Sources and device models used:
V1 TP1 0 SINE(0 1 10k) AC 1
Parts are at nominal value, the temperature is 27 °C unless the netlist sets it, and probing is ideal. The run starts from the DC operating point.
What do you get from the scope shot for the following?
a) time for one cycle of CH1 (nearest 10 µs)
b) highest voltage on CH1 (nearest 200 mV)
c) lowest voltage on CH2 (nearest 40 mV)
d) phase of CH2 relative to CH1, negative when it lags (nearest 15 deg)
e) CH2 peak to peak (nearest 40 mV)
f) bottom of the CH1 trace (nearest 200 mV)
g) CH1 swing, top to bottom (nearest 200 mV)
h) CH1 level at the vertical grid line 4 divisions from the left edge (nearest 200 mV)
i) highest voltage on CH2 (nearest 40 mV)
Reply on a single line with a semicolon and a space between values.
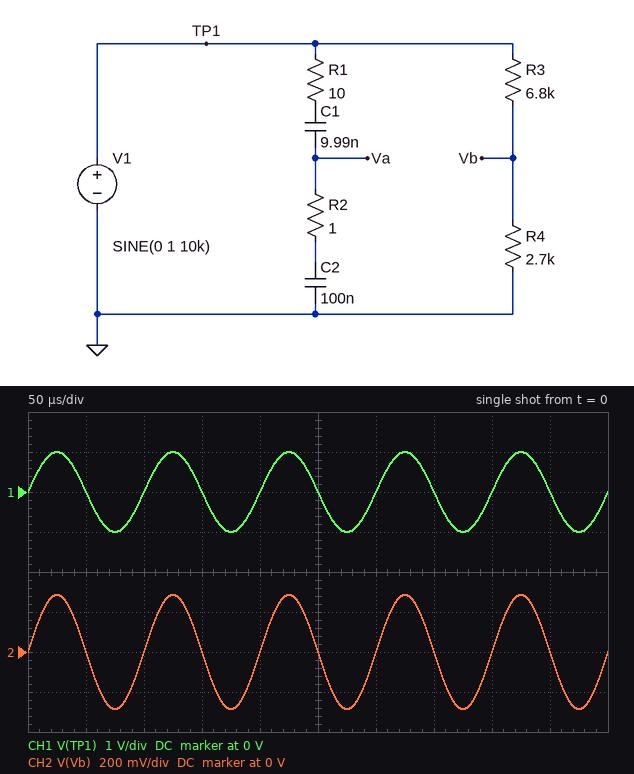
100 µs; 1.0 V; -280 mV; 0 deg; 560 mV; -1.0 V; 2.0 V; 0 V; 280 mV
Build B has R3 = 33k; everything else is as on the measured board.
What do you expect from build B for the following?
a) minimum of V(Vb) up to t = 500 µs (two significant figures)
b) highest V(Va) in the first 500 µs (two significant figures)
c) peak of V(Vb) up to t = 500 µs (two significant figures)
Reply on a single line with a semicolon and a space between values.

-76 mV; 91 mV; 76 mV
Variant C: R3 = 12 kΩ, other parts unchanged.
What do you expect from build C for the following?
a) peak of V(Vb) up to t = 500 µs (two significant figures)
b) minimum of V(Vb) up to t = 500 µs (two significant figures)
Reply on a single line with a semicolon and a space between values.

180 mV; -180 mV
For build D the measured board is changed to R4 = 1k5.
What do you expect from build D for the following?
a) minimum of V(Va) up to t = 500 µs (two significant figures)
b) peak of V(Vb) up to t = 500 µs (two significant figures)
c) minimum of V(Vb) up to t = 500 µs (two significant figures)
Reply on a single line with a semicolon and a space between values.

-91 mV; 180 mV; -180 mV
